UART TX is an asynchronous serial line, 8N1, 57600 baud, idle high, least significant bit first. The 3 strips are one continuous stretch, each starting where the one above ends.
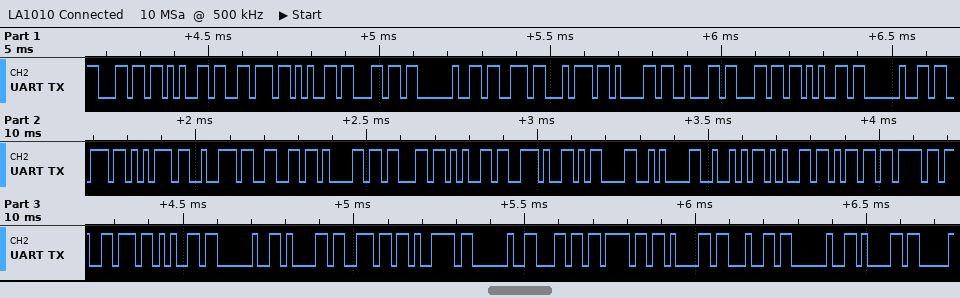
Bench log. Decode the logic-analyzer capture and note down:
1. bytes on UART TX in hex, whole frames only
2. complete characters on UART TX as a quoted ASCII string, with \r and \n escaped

0x6C 0x65 0x76 0x65 0x6C 0x20 0x73 0x74 0x61 0x62 0x6C 0x65 0x20 0x73 0x75 0x72 0x66 0x61 0x63 0x65 0x2E 0x0D 0x0A 0x52 0x65 0x6D 0x6F 0x76 0x65 0x20 0x61 0x6E 0x79 0x20 0x6C 0x6F 0x61 0x64 0x20 0x61
"level stable surface.\r\nRemove any load a"
